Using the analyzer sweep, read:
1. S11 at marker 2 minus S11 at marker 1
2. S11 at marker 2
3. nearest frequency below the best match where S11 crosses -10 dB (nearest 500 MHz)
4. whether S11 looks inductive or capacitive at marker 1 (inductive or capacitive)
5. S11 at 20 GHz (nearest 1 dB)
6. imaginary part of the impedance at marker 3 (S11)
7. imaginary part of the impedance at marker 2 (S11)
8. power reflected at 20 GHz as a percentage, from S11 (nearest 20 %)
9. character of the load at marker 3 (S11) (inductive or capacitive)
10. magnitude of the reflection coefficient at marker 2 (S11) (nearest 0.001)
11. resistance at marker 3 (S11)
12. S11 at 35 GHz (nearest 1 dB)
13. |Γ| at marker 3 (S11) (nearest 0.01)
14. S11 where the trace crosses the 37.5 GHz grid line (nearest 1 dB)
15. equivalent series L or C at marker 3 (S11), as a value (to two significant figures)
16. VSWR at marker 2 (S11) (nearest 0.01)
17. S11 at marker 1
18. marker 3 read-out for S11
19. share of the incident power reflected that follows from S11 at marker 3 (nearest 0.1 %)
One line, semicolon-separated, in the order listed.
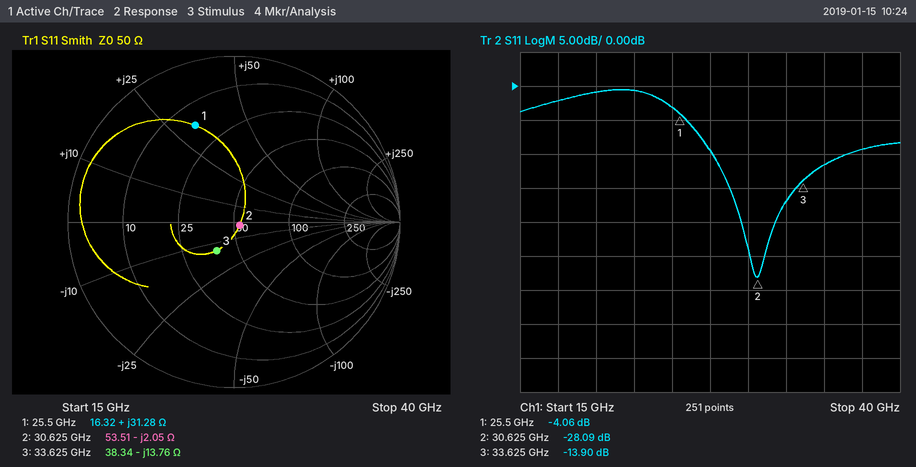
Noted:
-24.03 dB; -28.09 dB; 27.5 GHz; inductive; -1 dB; -13.76 Ω; -2.05 Ω; 80 %; capacitive; 0.039; 38.34 Ω; -12 dB; 0.20; -9 dB; 340 fF; 1.08; -4.06 dB; -13.90 dB; 4.1 %
